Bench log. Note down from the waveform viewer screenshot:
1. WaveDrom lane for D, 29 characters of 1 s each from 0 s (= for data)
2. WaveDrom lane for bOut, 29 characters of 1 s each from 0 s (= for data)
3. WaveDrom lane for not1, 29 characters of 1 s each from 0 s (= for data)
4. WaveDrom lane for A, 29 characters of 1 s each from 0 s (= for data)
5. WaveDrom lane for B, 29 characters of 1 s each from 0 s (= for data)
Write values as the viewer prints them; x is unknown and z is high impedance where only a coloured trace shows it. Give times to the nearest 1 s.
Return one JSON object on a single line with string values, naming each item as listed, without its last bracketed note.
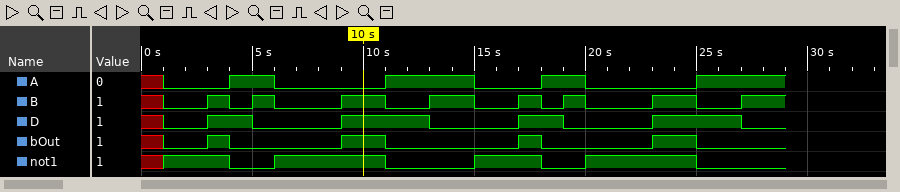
{"WaveDrom lane for D, 29 characters of 1 s each from 0 s": "{name: 'D', wave: 'x0.1.0...1...0...1.0...1...0.'}", "WaveDrom lane for bOut, 29 characters of 1 s each from 0 s": "{name: 'bOut', wave: 'x0.10....1.0.....10....1.0...'}", "WaveDrom lane for not1, 29 characters of 1 s each from 0 s": "{name: 'not1', wave: 'x1..0.1....0...1..0.1....0...'}", "WaveDrom lane for A, 29 characters of 1 s each from 0 s": "{name: 'A', wave: 'x0..1.0....1...0..1.0....1...'}", "WaveDrom lane for B, 29 characters of 1 s each from 0 s": "{name: 'B', wave: 'x0.1010..1.0.1.0.1010..1.0.1.'}"}
